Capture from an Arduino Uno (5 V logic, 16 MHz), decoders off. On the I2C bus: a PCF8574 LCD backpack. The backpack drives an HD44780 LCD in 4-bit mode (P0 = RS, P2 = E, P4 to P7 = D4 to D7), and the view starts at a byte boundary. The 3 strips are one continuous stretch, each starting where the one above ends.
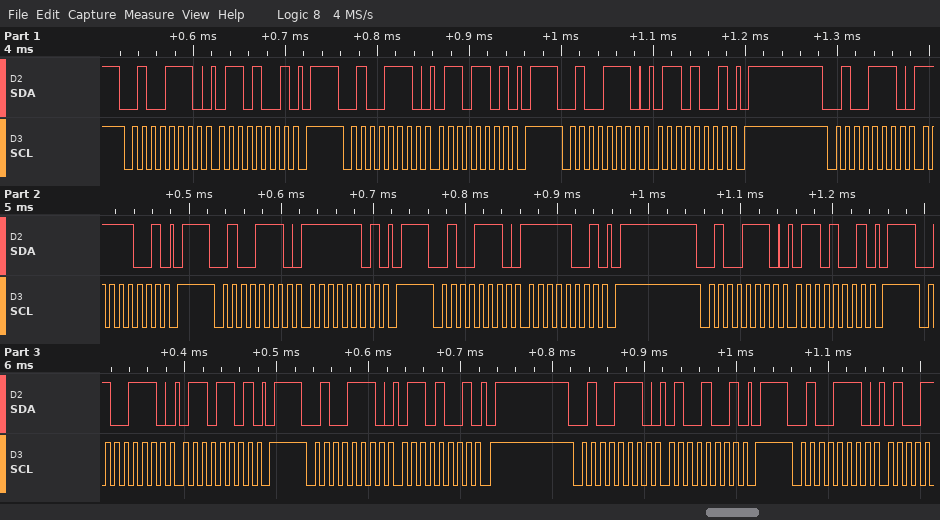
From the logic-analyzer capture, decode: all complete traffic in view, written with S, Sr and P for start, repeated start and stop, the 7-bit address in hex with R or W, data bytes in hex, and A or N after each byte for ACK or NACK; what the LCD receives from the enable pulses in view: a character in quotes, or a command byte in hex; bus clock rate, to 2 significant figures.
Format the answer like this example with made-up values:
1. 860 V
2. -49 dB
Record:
1. S 27W A 69 A P S 27W A 6D A P S 27W A 69 A P S 27W A F9 A P S 27W A FD A P S 27W A F9 A P S 27W A 69 A P S 27W A 6D A P S 27W A 69 A P S 27W A 49 A P S 27W A
2. 'o'
3. 100 kHz
